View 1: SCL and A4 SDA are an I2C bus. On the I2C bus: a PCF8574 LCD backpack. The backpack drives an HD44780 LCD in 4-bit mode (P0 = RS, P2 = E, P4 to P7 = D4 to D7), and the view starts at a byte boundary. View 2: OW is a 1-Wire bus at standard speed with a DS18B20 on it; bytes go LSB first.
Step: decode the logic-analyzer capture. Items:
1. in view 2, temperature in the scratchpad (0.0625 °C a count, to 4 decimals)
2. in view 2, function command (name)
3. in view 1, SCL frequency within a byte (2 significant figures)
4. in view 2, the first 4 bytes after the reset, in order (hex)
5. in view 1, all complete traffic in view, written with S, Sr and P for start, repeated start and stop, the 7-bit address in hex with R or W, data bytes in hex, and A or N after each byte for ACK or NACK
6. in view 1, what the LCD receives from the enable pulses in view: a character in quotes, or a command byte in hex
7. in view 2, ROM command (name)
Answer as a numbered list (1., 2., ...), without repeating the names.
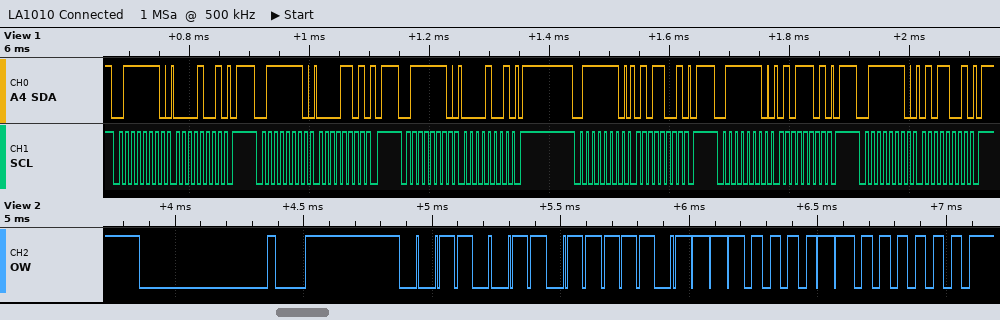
1. 24.4375 °C
2. Read Scratchpad
3. 100 kHz
4. CC BE 87 01
5. S 3FW A 09 A P S 3FW A 0D A P S 3FW A 09 A P S 3FW A 59 A P S 3FW A 5D A P S 3FW A 59 A P
6. data 0x05
7. Skip ROM
